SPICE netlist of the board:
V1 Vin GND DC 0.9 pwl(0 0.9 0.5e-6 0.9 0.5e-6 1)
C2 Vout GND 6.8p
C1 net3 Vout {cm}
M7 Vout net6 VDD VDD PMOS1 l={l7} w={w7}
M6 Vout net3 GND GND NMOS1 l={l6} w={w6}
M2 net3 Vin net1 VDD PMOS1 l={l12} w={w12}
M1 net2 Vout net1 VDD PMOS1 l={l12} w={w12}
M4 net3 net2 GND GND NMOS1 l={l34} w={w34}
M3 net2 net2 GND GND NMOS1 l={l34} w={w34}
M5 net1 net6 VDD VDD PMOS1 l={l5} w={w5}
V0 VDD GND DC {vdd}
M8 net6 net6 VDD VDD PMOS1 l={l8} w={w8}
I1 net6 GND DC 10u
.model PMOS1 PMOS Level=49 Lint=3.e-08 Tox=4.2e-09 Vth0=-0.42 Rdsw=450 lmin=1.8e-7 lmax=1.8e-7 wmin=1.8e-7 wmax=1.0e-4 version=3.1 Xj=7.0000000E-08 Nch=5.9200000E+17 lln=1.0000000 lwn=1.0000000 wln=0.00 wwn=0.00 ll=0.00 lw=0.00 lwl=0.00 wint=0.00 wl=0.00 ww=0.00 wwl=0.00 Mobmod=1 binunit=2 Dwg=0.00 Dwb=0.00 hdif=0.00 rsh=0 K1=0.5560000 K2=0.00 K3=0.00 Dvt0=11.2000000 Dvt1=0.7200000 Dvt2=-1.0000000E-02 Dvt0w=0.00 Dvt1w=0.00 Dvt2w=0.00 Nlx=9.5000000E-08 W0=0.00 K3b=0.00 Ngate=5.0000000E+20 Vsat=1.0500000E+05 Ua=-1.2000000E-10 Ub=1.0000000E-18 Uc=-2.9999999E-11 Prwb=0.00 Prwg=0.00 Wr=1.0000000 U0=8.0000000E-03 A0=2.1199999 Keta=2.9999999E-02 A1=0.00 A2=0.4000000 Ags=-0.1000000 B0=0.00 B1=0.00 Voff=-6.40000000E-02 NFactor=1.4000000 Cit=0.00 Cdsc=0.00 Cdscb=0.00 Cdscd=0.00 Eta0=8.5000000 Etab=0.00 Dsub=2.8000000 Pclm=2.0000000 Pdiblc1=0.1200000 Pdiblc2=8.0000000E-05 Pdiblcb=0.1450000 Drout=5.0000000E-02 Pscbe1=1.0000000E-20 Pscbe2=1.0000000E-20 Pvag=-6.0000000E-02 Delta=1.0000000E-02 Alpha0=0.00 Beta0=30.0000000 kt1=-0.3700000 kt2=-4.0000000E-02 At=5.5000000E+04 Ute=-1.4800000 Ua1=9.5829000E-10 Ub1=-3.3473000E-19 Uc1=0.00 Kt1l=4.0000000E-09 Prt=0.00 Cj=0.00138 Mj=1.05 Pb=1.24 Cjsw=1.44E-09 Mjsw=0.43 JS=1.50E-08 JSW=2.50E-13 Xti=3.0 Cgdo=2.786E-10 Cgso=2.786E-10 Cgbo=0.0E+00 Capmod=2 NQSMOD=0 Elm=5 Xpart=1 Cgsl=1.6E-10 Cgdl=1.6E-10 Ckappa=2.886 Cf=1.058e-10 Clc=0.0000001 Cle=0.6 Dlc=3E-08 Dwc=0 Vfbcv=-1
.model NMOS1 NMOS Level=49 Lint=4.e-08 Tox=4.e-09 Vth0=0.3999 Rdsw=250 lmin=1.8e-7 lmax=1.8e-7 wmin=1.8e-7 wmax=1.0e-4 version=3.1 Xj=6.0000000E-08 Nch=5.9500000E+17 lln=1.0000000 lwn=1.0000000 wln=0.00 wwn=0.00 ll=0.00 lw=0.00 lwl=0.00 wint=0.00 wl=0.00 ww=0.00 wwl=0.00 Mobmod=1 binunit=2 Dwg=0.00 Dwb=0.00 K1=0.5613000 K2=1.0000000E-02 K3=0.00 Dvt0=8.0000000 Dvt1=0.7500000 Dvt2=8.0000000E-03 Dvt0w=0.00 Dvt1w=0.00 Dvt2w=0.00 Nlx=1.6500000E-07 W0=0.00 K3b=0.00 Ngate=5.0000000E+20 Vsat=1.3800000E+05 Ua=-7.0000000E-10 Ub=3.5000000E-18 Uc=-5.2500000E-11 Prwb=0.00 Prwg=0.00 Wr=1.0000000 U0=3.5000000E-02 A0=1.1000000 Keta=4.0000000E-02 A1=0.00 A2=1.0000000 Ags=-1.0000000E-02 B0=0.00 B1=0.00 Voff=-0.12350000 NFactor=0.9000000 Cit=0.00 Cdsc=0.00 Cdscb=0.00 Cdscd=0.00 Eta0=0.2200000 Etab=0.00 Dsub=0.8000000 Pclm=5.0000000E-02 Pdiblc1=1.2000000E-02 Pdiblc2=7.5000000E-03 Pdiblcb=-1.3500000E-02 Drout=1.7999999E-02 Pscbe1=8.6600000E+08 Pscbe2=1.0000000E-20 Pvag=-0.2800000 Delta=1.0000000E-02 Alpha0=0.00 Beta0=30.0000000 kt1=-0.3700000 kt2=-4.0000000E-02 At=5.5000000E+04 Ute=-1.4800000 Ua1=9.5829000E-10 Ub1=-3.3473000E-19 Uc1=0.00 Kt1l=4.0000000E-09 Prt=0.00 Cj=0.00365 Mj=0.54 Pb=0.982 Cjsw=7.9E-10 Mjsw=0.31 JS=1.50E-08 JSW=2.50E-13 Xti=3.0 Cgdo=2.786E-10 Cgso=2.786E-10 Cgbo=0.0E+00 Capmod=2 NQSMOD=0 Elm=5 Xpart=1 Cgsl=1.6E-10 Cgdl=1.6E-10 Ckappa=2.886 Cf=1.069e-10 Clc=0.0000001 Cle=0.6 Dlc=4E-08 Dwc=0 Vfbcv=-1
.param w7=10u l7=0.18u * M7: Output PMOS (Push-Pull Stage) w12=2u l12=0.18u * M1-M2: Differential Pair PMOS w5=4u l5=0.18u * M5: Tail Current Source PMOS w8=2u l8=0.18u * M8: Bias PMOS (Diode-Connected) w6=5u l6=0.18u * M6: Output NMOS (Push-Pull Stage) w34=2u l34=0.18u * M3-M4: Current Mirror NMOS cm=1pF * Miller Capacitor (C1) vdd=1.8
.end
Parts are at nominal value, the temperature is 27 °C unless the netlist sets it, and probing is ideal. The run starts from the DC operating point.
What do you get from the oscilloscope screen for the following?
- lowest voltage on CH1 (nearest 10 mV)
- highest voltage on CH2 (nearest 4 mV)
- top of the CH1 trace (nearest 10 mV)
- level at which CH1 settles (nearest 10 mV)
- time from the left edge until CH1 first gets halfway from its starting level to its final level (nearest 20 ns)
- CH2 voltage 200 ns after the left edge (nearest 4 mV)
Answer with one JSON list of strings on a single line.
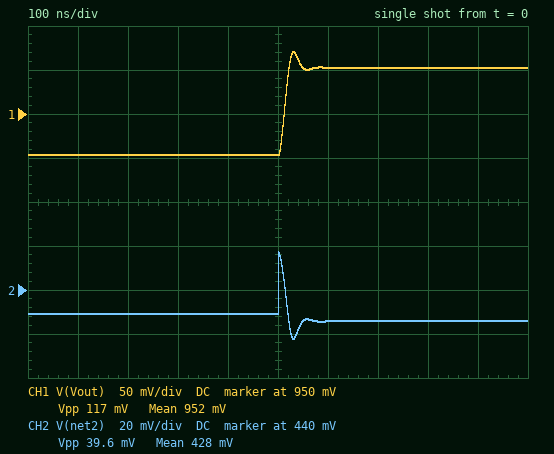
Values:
["900 mV", "456 mV", "1.02 V", "1.00 V", "520 ns", "428 mV"]
